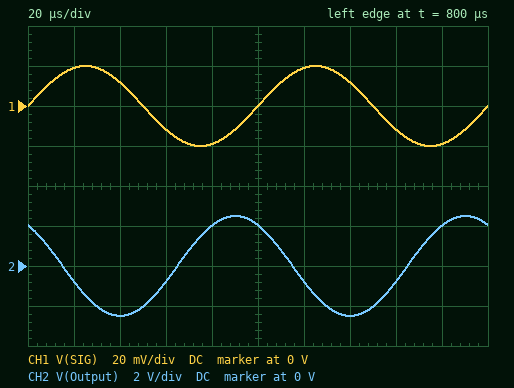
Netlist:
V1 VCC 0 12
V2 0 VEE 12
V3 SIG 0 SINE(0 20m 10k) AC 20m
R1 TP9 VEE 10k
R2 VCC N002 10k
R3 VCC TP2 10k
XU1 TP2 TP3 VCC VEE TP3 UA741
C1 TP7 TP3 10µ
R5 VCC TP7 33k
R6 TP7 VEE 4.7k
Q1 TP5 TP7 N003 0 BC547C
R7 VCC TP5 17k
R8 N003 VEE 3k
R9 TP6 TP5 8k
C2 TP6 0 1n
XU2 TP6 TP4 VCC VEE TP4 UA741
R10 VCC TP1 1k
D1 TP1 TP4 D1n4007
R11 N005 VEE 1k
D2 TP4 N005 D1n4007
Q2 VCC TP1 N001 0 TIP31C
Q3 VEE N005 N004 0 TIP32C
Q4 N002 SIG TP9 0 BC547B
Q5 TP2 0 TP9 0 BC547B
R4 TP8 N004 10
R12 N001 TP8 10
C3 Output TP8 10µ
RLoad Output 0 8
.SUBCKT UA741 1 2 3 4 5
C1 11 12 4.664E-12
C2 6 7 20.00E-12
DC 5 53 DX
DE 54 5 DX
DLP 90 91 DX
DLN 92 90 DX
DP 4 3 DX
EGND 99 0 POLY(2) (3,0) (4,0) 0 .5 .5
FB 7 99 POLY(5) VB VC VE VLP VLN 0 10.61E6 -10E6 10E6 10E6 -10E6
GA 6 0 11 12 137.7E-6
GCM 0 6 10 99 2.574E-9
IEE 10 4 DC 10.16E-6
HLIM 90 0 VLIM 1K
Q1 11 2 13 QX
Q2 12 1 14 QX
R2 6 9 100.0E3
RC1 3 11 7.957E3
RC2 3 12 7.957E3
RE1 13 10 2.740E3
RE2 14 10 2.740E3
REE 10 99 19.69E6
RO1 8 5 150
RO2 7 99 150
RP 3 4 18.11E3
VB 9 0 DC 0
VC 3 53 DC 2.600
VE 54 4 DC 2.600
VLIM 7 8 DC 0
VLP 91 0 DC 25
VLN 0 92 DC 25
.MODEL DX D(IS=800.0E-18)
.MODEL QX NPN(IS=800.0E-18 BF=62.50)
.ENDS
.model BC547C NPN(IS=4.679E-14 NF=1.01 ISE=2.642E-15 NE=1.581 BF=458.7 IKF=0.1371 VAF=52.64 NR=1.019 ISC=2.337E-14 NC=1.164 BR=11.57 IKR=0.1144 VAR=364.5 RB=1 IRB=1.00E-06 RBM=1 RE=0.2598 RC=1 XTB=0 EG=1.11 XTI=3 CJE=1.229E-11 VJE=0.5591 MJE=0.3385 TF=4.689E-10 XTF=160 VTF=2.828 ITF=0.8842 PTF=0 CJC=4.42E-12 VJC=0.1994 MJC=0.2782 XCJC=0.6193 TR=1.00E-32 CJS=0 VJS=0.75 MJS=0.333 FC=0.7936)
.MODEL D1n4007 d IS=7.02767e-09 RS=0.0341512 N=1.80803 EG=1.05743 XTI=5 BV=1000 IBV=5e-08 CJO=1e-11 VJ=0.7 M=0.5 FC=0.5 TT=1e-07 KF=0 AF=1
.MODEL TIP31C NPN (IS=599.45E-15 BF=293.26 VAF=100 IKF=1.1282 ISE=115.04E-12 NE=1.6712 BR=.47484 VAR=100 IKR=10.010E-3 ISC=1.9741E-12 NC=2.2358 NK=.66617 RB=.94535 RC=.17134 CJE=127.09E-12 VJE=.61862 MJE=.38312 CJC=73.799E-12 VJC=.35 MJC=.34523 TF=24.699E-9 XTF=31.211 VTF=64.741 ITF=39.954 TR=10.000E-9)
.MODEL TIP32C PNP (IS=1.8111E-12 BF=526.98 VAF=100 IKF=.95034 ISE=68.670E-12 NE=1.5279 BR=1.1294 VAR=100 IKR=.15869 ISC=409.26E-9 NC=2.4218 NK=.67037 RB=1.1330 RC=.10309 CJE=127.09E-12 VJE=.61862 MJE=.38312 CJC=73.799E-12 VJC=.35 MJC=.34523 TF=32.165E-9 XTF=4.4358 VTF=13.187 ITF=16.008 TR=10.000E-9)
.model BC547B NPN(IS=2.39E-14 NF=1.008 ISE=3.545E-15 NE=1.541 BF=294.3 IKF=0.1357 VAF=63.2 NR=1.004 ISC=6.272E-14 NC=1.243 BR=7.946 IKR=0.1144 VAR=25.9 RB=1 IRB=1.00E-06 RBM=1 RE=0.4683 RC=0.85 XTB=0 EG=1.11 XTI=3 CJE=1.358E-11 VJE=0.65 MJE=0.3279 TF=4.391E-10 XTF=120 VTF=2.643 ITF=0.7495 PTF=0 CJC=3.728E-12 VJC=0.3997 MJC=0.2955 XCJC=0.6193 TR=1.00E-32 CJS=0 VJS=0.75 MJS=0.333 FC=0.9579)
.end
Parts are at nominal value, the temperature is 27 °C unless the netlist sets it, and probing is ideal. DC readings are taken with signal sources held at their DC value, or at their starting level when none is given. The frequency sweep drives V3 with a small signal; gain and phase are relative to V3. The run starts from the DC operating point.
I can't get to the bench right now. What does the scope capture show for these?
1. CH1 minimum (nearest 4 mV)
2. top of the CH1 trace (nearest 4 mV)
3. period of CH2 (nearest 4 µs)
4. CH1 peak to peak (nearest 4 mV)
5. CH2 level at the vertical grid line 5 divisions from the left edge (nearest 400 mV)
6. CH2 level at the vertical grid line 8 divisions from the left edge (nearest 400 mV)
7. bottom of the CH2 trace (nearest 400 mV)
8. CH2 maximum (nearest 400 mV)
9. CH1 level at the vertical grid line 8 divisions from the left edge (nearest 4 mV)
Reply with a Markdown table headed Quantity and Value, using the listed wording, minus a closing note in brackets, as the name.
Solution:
| Quantity | Value |
|---|---|
| CH1 minimum | -20 mV |
| top of the CH1 trace | 20 mV |
| period of CH2 | 100 µs |
| CH1 peak to peak | 40 mV |
| CH2 level at the vertical grid line 5 divisions from the left edge | 2.0 V |
| CH2 level at the vertical grid line 8 divisions from the left edge | -800 mV |
| bottom of the CH2 trace | -2.4 V |
| CH2 maximum | 2.4 V |
| CH1 level at the vertical grid line 8 divisions from the left edge | -12 mV |
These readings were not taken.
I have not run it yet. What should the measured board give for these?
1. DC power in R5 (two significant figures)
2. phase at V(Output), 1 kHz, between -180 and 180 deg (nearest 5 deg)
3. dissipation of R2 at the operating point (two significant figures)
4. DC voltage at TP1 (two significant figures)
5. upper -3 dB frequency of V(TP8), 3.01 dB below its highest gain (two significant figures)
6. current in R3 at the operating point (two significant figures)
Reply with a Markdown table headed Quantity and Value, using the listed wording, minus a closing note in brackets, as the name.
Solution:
| Quantity | Value |
|---|---|
| DC power in R5 | 13 mW |
| phase at V(Output), 1 kHz, between -180 and 180 deg | -140 deg |
| dissipation of R2 at the operating point | 3.2 mW |
| DC voltage at TP1 | -750 mV |
| upper -3 dB frequency of V(TP8), 3.01 dB below its highest gain | 1.6 kHz |
| current in R3 at the operating point | 570 µA |
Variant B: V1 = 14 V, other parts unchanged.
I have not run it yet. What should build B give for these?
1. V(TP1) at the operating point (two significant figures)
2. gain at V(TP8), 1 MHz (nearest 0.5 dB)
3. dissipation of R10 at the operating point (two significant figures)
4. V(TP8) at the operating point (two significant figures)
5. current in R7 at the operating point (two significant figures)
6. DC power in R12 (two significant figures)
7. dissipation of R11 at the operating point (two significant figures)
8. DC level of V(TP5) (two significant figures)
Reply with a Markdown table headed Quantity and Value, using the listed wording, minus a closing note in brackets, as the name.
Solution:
| Quantity | Value |
|---|---|
| V(TP1) at the operating point | -140 mV |
| gain at V(TP8), 1 MHz | 0.5 dB |
| dissipation of R10 at the operating point | 200 mW |
| V(TP8) at the operating point | -830 mV |
| current in R7 at the operating point | 870 µA |
| DC power in R12 | 710 µW |
| dissipation of R11 at the operating point | 110 mW |
| DC level of V(TP5) | -820 mV |
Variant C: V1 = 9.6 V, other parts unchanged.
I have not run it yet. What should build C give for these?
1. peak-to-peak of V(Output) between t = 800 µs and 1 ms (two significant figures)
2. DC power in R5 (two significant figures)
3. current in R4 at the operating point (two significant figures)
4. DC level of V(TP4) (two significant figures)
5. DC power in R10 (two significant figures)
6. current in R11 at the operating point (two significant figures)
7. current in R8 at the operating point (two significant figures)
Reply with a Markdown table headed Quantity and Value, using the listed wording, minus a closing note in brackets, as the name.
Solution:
| Quantity | Value |
|---|---|
| peak-to-peak of V(Output) between t = 800 µs and 1 ms | 4.9 V |
| DC power in R5 | 11 mW |
| current in R4 at the operating point | 7.7 mA |
| DC level of V(TP4) | -2.2 V |
| DC power in R10 | 120 mW |
| current in R11 at the operating point | 9.2 mA |
| current in R8 at the operating point | 690 µA |
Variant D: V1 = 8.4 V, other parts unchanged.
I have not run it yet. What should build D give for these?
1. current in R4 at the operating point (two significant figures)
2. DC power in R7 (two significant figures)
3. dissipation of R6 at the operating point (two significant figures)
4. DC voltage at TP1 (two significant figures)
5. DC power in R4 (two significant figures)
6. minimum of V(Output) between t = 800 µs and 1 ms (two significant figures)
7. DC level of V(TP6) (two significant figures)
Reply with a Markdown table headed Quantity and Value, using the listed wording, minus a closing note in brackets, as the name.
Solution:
| Quantity | Value |
|---|---|
| current in R4 at the operating point | 7.5 mA |
| DC power in R7 | 7.0 mW |
| dissipation of R6 at the operating point | 1.4 mW |
| DC voltage at TP1 | -1.9 V |
| DC power in R4 | 560 µW |
| minimum of V(Output) between t = 800 µs and 1 ms | -2.4 V |
| DC level of V(TP6) | -2.5 V |
